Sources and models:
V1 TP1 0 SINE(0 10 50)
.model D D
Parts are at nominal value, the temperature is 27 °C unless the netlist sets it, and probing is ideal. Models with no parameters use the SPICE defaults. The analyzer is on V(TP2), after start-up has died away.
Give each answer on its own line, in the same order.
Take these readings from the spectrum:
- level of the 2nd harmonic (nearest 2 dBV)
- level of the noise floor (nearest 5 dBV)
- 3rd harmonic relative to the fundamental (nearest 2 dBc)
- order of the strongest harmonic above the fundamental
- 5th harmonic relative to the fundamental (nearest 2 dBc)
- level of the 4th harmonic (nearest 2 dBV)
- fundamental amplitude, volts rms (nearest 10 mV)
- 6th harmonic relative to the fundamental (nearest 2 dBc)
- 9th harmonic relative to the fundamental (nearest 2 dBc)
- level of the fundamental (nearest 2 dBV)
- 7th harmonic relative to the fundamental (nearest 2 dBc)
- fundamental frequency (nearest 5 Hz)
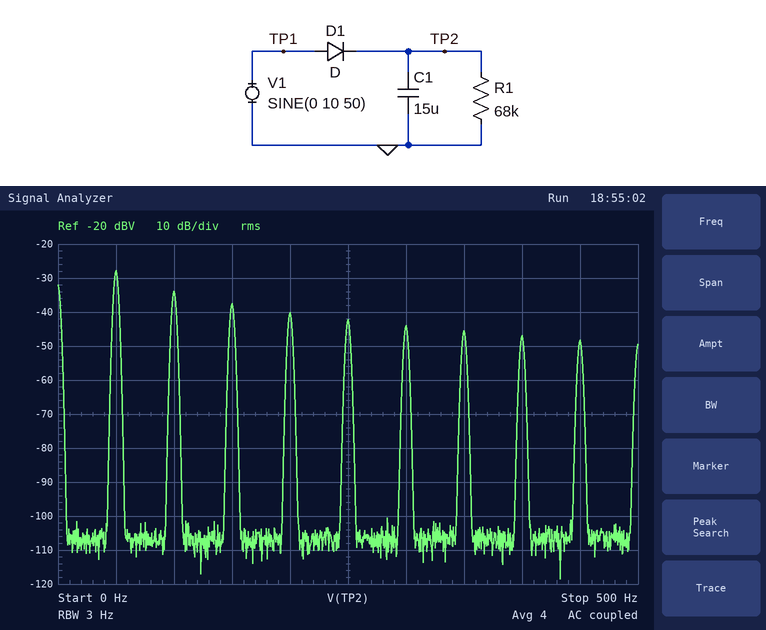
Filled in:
-34 dBV
-105 dBV
-10 dBc
2
-14 dBc
-40 dBV
40 mV
-16 dBc
-20 dBc
-28 dBV
-18 dBc
50 Hz
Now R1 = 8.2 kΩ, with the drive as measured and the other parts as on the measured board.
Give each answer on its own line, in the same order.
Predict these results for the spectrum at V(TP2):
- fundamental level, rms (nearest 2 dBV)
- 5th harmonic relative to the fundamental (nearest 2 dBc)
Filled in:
-10 dBV
-16 dBc
